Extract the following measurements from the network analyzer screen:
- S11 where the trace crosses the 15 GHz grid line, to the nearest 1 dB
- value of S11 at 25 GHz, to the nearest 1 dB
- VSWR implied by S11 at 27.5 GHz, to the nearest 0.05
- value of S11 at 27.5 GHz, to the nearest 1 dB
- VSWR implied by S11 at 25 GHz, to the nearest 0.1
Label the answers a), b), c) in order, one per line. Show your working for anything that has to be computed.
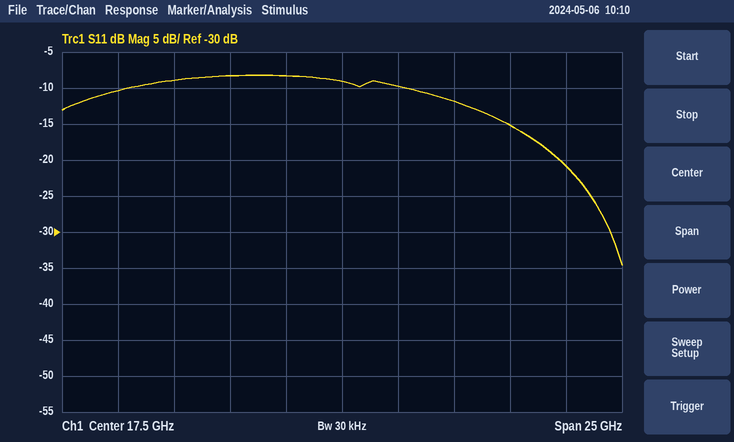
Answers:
a) -8 dB
b) -15 dB
c) |Γ| = 10^(-21/20) = 0.0891; VSWR = (1 + 0.0891)/(1 − 0.0891) ≈ 1.20
d) -21 dB
e) |Γ| = 10^(-15/20) = 0.1778; VSWR = (1 + 0.1778)/(1 − 0.1778) ≈ 1.4
